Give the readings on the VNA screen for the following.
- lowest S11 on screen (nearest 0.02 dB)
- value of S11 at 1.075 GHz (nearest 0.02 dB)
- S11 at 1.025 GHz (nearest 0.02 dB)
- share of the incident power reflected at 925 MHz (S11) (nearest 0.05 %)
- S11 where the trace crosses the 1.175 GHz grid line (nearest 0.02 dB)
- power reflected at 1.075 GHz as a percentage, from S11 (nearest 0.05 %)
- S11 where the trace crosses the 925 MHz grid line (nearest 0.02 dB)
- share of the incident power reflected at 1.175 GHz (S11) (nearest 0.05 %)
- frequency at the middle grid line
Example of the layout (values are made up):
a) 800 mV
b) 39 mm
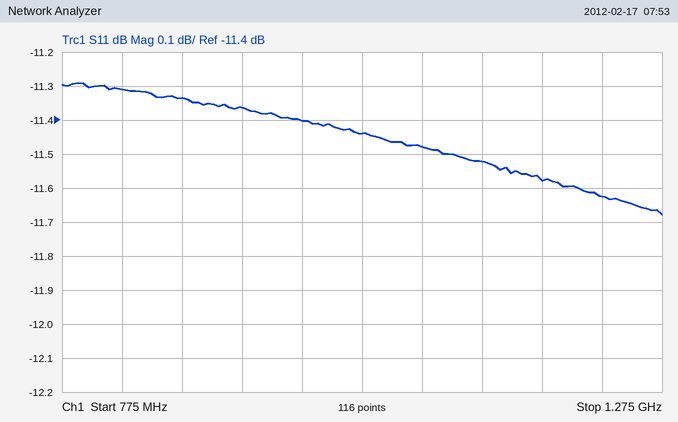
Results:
a) -11.68 dB
b) -11.48 dB
c) -11.44 dB
d) 7.30 %
e) -11.58 dB
f) 7.10 %
g) -11.36 dB
h) 6.95 %
i) 1.025 GHz
